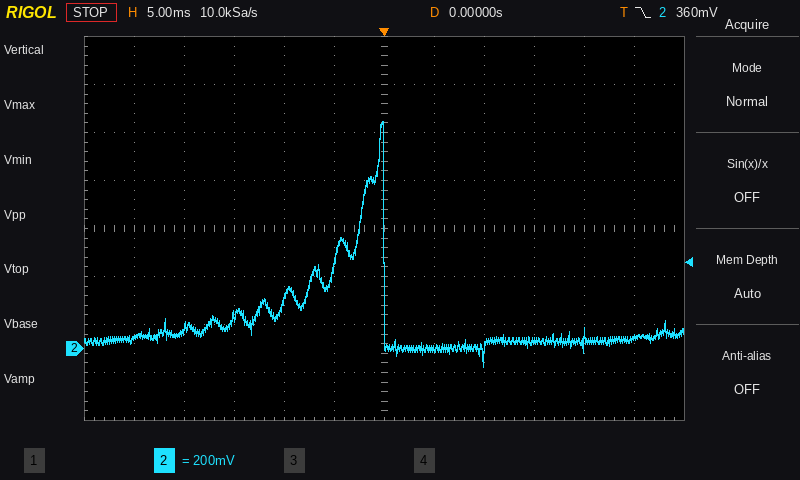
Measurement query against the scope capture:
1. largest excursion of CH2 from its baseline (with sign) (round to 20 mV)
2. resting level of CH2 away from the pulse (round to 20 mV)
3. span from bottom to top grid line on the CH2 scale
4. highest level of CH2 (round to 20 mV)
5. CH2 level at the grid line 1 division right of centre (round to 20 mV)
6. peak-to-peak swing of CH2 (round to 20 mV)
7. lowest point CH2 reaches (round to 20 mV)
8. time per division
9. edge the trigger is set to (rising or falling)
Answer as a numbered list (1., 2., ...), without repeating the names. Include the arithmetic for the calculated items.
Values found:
1. 940 mV − (40 mV) = +900 mV
2. 40 mV
3. 1.6 V
4. 940 mV
5. 0 mV
6. 940 mV − (-80 mV) = 1.02 V
7. -80 mV
8. 5 ms
9. falling
